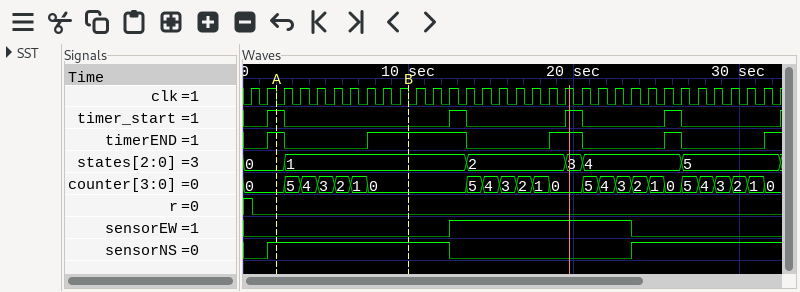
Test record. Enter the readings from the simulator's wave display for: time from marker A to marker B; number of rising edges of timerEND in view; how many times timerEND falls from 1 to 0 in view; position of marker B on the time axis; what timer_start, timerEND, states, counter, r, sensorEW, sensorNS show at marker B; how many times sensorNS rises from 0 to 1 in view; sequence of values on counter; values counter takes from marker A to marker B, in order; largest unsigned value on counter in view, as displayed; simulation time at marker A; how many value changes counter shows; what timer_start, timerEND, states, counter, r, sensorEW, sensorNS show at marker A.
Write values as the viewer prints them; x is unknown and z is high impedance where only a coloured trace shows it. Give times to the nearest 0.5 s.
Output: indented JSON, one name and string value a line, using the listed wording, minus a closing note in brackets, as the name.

{
  "time from marker A to marker B": "8 s",
  "number of rising edges of timerEND in view": "5",
  "how many times timerEND falls from 1 to 0 in view": "4",
  "position of marker B on the time axis": "10 s",
  "what timer_start, timerEND, states, counter, r, sensorEW, sensorNS show at marker B": "timer_start=0, timerEND=1, states=1, counter=0, r=0, sensorEW=0, sensorNS=1",
  "how many times sensorNS rises from 0 to 1 in view": "2",
  "sequence of values on counter": "0, 5, 4, 3, 2, 1, 0, 5, 4, 3, 2, 1, 0, 5, 4, 3, 2, 1, 0, 5, 4, 3, 2, 1, 0",
  "values counter takes from marker A to marker B, in order": "0, 5, 4, 3, 2, 1, 0",
  "largest unsigned value on counter in view, as displayed": "5",
  "simulation time at marker A": "2 s",
  "how many value changes counter shows": "24",
  "what timer_start, timerEND, states, counter, r, sensorEW, sensorNS show at marker A": "timer_start=1, timerEND=1, states=0, counter=0, r=0, sensorEW=0, sensorNS=1"
}
